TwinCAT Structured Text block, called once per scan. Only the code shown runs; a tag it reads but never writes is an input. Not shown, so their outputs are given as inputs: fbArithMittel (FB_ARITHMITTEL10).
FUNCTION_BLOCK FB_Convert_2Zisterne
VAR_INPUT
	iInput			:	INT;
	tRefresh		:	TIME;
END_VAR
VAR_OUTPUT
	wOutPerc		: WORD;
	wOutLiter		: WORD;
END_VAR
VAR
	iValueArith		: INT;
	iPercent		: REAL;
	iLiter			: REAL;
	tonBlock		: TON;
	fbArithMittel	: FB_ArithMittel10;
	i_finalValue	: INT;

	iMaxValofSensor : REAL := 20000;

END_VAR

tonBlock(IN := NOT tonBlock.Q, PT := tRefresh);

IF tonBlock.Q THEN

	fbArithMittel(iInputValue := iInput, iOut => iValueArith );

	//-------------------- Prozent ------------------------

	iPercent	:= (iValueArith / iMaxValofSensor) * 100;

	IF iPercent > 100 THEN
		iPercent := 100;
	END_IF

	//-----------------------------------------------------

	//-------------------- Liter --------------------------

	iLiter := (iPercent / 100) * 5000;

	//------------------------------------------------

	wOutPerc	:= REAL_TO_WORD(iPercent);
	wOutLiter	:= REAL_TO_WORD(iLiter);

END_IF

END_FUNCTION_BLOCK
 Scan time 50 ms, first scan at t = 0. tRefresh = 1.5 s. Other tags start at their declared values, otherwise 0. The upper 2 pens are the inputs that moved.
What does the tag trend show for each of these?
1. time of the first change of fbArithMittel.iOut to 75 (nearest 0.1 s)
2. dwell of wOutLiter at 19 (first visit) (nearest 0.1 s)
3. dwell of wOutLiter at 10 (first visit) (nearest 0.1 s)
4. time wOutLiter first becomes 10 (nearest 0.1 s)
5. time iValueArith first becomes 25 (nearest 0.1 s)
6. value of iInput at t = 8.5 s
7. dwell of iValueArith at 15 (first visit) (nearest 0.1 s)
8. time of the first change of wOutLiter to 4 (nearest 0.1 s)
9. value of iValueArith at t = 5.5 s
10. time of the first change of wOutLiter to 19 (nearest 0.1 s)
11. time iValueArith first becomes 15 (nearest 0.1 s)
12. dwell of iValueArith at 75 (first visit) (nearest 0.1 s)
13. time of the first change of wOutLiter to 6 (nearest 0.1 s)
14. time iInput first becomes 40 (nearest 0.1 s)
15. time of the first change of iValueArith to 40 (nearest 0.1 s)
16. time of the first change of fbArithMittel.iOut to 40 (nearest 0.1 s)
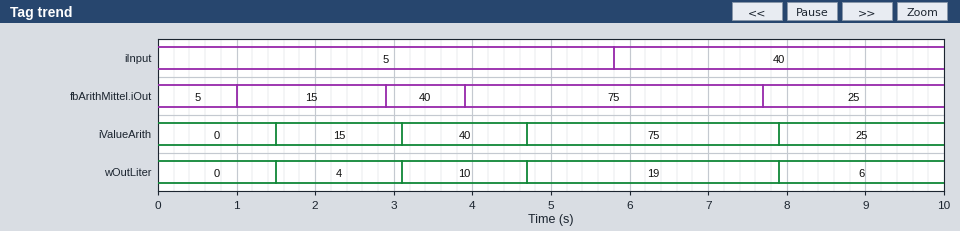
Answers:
3.9 s
3.2 s
1.6 s
3.1 s
7.9 s
40
1.6 s
1.5 s
75
4.7 s
1.5 s
3.2 s
7.9 s
5.8 s
3.1 s
2.9 s
